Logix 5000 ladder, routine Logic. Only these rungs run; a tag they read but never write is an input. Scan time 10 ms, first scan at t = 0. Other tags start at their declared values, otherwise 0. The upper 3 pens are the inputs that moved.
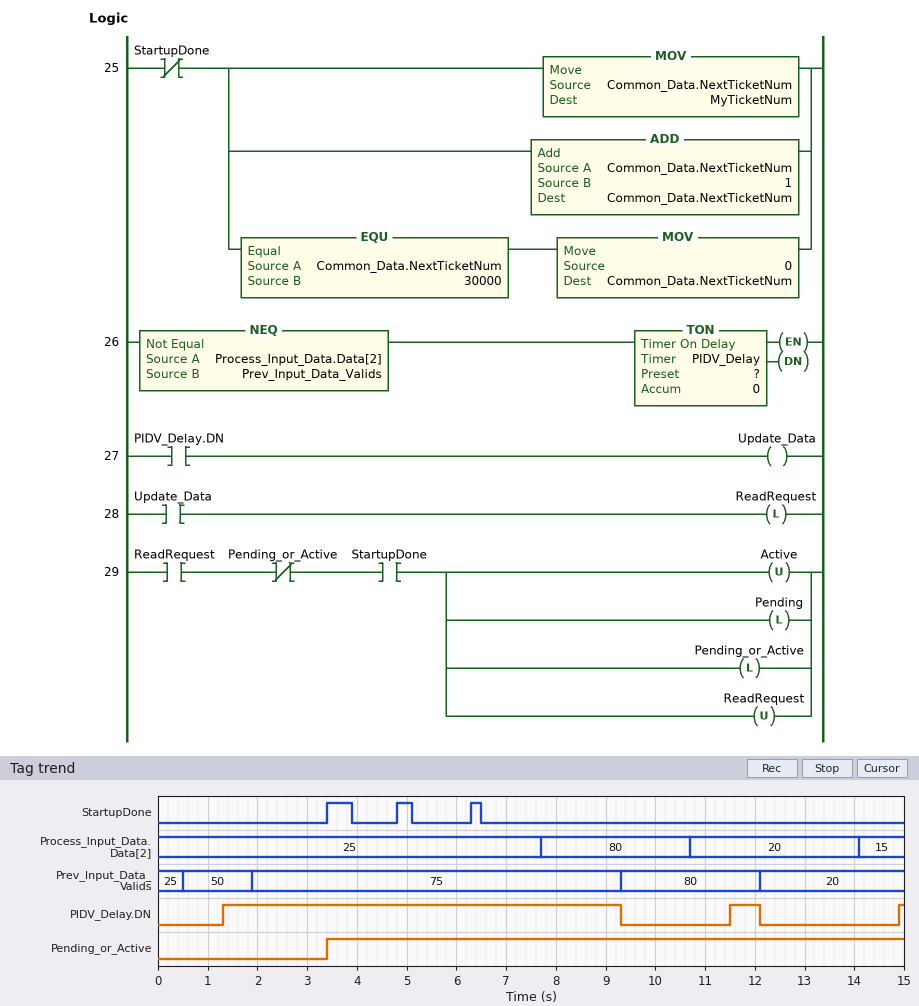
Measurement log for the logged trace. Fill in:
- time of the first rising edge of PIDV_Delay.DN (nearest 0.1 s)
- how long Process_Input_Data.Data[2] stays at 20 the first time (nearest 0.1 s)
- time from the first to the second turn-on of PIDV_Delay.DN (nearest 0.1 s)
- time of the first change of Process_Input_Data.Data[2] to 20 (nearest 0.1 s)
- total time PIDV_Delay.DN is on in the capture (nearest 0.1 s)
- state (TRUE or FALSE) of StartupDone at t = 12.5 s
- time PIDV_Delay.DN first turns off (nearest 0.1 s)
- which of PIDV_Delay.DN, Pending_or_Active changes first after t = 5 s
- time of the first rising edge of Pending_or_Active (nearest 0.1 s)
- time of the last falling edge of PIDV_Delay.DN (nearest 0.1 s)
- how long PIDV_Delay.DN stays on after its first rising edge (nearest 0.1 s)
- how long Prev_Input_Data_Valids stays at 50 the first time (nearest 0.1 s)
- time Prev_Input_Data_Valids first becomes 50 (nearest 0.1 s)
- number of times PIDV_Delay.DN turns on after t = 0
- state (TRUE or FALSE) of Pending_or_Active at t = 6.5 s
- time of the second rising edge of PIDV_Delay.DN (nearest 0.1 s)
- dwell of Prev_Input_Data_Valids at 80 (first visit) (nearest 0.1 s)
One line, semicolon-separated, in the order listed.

1.3 s; 3.4 s; 10.2 s; 10.7 s; 8.7 s; FALSE; 9.3 s; PIDV_Delay.DN; 3.4 s; 12.1 s; 8.0 s; 1.4 s; 0.5 s; 3; TRUE; 11.5 s; 2.8 s
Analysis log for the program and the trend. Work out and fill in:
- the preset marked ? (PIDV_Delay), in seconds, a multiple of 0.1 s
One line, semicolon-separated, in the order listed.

0.8 s
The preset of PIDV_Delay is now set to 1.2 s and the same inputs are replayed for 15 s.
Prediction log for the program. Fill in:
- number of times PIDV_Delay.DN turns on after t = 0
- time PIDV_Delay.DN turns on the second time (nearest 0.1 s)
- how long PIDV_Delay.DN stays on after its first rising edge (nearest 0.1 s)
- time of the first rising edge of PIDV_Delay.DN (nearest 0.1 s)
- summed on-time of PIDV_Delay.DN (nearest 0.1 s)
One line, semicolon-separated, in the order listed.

2; 11.9 s; 7.6 s; 1.7 s; 7.8 s
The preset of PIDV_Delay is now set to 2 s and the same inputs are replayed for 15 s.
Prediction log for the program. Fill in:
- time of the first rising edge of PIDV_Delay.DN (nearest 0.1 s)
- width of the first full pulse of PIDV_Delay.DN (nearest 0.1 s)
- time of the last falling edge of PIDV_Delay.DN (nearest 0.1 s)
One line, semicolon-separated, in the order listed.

2.5 s; 6.8 s; 9.3 s
